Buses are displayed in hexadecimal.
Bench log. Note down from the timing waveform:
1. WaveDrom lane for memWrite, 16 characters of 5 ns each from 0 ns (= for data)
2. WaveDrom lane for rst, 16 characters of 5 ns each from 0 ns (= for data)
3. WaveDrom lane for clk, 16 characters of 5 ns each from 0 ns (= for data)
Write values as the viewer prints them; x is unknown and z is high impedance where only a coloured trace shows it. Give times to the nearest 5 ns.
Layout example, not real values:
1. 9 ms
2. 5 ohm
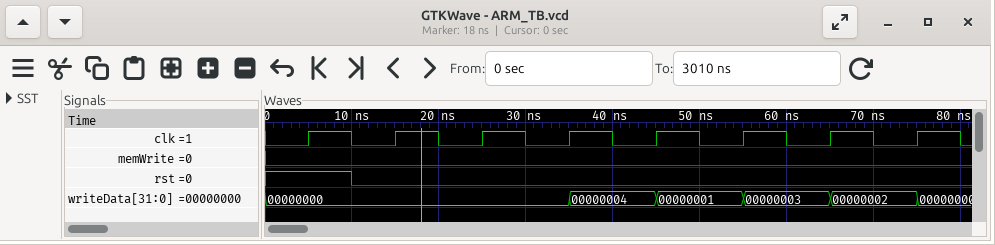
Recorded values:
1. {name: 'memWrite', wave: '0...............'}
2. {name: 'rst', wave: '1.0.............'}
3. {name: 'clk', wave: '0101010101010101'}
